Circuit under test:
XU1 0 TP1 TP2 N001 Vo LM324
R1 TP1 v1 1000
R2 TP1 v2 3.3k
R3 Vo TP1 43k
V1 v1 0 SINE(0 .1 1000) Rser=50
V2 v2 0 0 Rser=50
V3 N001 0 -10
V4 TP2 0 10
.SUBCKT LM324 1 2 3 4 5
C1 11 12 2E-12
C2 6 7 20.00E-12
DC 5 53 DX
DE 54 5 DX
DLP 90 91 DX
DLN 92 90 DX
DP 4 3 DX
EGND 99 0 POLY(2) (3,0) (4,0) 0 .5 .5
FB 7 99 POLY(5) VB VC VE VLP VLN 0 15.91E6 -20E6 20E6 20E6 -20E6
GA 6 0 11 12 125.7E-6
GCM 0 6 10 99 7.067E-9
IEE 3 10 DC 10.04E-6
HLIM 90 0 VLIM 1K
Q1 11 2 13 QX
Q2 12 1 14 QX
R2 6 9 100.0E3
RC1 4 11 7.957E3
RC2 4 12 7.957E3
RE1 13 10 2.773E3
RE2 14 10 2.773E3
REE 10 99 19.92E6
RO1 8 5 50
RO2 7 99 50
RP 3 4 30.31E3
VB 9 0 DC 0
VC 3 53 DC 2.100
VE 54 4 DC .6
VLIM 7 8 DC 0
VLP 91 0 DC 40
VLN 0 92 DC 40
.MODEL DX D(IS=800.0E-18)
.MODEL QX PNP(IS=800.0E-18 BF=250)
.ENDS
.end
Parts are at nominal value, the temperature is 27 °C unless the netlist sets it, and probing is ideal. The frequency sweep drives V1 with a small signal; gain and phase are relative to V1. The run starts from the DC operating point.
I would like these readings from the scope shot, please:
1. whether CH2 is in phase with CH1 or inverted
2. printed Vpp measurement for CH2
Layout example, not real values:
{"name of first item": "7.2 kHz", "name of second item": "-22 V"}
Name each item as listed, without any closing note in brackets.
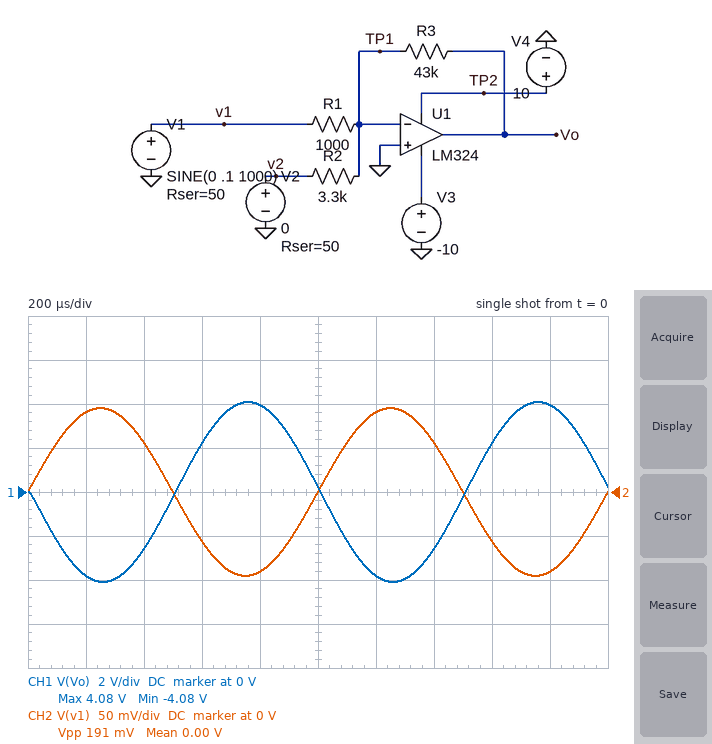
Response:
{"whether CH2 is in phase with CH1 or inverted": "inverted", "printed Vpp measurement for CH2": "191 mV"}
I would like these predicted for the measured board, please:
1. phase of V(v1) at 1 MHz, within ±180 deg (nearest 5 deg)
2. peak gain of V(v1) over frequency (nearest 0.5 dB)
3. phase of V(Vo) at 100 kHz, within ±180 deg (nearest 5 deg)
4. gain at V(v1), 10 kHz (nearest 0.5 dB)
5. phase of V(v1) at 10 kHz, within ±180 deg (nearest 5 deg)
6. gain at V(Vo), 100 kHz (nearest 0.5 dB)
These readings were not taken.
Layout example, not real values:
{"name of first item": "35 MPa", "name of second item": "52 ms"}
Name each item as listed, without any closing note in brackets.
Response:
{"phase of V(v1) at 1 MHz, within ±180 deg": "0 deg", "peak gain of V(v1) over frequency": "0 dB", "phase of V(Vo) at 100 kHz, within ±180 deg": "100 deg", "gain at V(v1), 10 kHz": "-0.5 dB", "phase of V(v1) at 10 kHz, within ±180 deg": "0 deg", "gain at V(Vo), 100 kHz": "17.5 dB"}
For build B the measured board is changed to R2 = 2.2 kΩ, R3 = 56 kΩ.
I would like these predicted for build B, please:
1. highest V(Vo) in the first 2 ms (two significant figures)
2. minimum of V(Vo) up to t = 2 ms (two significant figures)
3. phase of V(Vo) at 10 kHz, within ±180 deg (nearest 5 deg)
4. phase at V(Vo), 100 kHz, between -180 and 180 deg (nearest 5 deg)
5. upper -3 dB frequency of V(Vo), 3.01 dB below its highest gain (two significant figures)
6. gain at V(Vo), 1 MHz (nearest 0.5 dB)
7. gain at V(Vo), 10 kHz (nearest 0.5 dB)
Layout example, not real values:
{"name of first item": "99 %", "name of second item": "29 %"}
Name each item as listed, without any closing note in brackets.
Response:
{"highest V(Vo) in the first 2 ms": "5.3 V", "minimum of V(Vo) up to t = 2 ms": "-5.3 V", "phase of V(Vo) at 10 kHz, within ±180 deg": "140 deg", "phase at V(Vo), 100 kHz, between -180 and 180 deg": "95 deg", "upper -3 dB frequency of V(Vo), 3.01 dB below its highest gain": "13 kHz", "gain at V(Vo), 1 MHz": "-3.5 dB", "gain at V(Vo), 10 kHz": "32.5 dB"}
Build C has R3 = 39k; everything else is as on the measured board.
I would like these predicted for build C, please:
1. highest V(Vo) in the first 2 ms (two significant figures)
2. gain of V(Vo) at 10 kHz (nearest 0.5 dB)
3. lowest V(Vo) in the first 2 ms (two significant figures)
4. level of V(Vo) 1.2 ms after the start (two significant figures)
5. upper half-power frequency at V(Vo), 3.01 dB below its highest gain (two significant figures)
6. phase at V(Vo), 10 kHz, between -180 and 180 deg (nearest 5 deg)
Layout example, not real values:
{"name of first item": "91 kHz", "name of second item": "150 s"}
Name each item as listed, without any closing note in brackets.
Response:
{"highest V(Vo) in the first 2 ms": "3.7 V", "gain of V(Vo) at 10 kHz": "30.5 dB", "lowest V(Vo) in the first 2 ms": "-3.7 V", "level of V(Vo) 1.2 ms after the start": "-3.5 V", "upper half-power frequency at V(Vo), 3.01 dB below its highest gain": "20 kHz", "phase at V(Vo), 10 kHz, between -180 and 180 deg": "155 deg"}
